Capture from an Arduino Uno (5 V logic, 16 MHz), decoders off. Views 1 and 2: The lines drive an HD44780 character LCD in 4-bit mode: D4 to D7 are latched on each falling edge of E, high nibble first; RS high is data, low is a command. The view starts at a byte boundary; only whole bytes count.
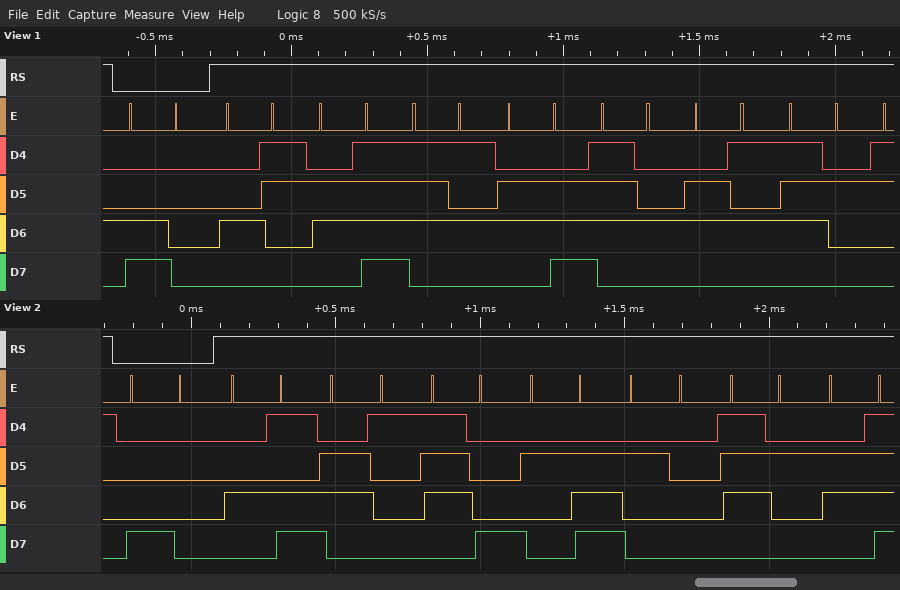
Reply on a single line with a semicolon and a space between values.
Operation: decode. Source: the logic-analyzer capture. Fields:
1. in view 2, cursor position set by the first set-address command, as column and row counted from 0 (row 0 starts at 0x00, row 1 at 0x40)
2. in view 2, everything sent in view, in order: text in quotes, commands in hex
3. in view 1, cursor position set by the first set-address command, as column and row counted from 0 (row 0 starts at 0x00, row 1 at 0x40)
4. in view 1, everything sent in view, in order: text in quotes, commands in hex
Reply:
column 0, row 0; 0x80 "Max. ro"; column 0, row 1; 0xC0 "Counter"
